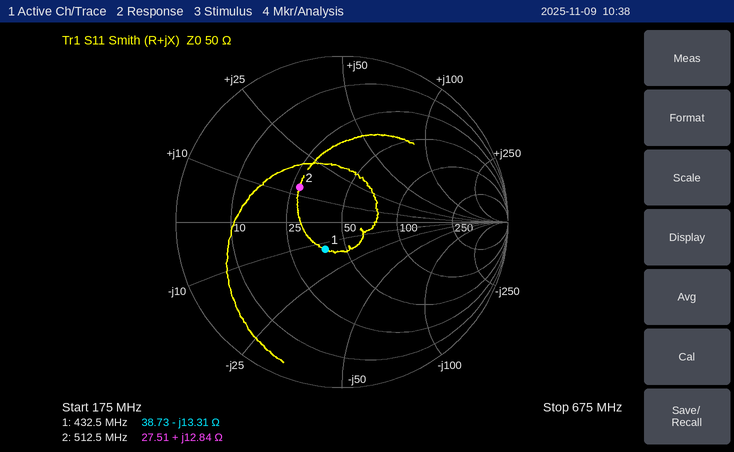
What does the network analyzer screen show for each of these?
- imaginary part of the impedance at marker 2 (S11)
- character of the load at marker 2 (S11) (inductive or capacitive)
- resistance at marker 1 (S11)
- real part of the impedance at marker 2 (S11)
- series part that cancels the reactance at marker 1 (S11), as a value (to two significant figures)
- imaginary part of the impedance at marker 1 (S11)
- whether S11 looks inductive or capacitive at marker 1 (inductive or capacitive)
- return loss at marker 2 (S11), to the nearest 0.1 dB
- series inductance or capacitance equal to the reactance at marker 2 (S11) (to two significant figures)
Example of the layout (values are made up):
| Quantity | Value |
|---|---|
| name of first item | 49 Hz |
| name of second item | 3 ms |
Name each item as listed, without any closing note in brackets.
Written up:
| Quantity | Value |
|---|---|
| imaginary part of the impedance at marker 2 | +12.84 Ω |
| character of the load at marker 2 (S11) | inductive |
| resistance at marker 1 | 38.73 Ω |
| real part of the impedance at marker 2 | 27.51 Ω |
| series part that cancels the reactance at marker 1 (S11), as a value | 4.9 nH |
| imaginary part of the impedance at marker 1 | -13.31 Ω |
| whether S11 looks inductive or capacitive at marker 1 | capacitive |
| return loss at marker 2 (S11), to the nearest 0.1 dB | 9.6 dB |
| series inductance or capacitance equal to the reactance at marker 2 (S11) | 4.0 nH |
